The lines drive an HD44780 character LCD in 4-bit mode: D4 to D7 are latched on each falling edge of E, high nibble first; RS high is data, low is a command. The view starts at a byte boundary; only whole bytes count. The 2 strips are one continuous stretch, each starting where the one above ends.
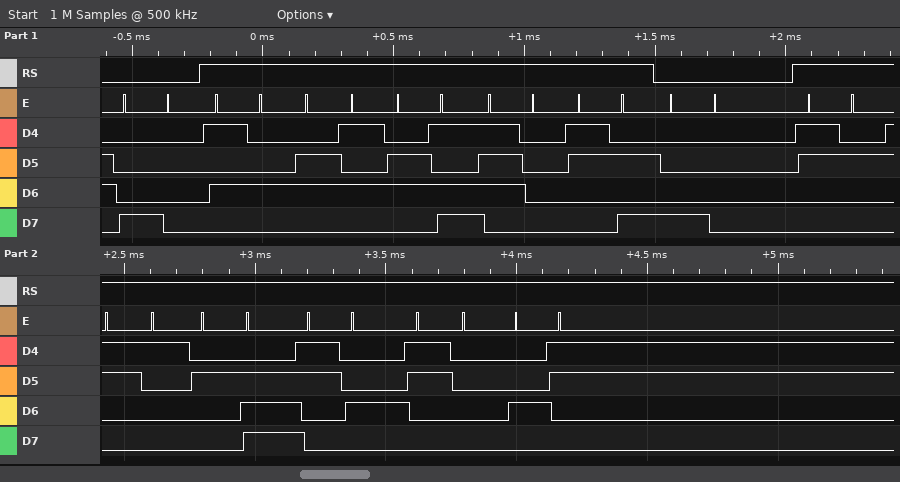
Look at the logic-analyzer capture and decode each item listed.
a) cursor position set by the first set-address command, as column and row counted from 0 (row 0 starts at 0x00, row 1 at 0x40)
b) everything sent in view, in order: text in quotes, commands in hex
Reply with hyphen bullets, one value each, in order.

- column 0, row 0
- 0x80 "Temp:" 0x80 "21.40C"
